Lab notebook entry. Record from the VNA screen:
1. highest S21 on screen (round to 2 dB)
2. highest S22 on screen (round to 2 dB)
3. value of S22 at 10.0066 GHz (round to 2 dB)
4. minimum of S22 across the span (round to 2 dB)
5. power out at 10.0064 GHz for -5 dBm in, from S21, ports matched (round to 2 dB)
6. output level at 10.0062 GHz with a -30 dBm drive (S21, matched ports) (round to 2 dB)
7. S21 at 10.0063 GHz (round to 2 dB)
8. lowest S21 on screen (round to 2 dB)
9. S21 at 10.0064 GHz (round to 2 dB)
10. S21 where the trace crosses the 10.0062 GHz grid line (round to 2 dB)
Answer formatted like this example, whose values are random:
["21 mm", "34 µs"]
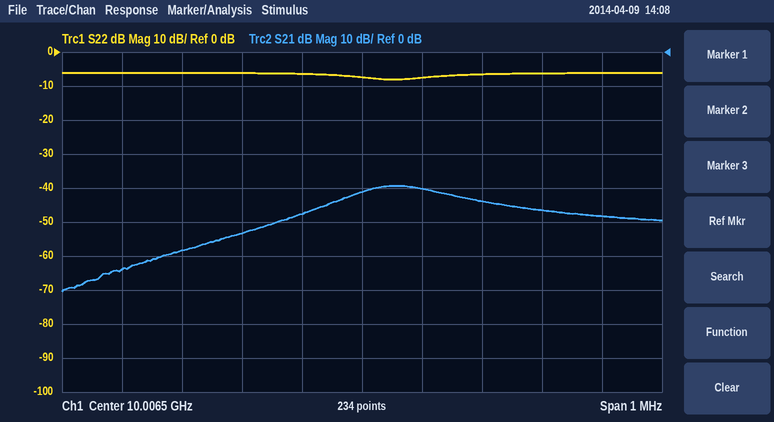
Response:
["-40 dB", "-6 dB", "-8 dB", "-8 dB", "-52 dBm", "-88 dBm", "-54 dB", "-70 dB", "-48 dB", "-58 dB"]
